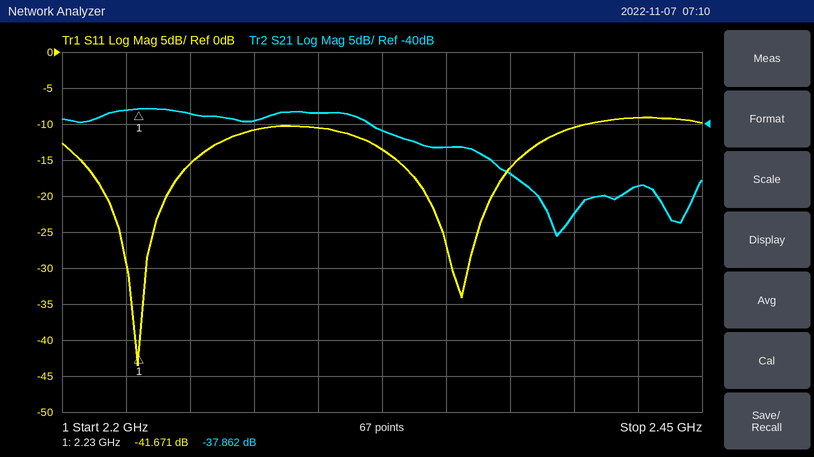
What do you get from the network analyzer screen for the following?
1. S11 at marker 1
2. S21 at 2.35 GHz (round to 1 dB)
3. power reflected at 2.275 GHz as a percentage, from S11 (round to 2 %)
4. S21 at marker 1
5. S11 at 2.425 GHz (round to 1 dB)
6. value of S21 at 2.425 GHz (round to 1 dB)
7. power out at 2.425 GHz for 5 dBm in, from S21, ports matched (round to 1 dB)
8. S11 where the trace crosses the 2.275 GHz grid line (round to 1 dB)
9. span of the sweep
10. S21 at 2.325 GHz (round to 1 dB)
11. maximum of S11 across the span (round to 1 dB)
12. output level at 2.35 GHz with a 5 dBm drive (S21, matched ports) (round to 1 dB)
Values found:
-41.671 dB
-43 dB
8 %
-37.862 dB
-9 dB
-49 dB
-44 dBm
-11 dB
250 MHz
-41 dB
-9 dB
-38 dBm
